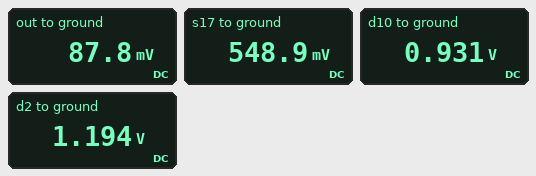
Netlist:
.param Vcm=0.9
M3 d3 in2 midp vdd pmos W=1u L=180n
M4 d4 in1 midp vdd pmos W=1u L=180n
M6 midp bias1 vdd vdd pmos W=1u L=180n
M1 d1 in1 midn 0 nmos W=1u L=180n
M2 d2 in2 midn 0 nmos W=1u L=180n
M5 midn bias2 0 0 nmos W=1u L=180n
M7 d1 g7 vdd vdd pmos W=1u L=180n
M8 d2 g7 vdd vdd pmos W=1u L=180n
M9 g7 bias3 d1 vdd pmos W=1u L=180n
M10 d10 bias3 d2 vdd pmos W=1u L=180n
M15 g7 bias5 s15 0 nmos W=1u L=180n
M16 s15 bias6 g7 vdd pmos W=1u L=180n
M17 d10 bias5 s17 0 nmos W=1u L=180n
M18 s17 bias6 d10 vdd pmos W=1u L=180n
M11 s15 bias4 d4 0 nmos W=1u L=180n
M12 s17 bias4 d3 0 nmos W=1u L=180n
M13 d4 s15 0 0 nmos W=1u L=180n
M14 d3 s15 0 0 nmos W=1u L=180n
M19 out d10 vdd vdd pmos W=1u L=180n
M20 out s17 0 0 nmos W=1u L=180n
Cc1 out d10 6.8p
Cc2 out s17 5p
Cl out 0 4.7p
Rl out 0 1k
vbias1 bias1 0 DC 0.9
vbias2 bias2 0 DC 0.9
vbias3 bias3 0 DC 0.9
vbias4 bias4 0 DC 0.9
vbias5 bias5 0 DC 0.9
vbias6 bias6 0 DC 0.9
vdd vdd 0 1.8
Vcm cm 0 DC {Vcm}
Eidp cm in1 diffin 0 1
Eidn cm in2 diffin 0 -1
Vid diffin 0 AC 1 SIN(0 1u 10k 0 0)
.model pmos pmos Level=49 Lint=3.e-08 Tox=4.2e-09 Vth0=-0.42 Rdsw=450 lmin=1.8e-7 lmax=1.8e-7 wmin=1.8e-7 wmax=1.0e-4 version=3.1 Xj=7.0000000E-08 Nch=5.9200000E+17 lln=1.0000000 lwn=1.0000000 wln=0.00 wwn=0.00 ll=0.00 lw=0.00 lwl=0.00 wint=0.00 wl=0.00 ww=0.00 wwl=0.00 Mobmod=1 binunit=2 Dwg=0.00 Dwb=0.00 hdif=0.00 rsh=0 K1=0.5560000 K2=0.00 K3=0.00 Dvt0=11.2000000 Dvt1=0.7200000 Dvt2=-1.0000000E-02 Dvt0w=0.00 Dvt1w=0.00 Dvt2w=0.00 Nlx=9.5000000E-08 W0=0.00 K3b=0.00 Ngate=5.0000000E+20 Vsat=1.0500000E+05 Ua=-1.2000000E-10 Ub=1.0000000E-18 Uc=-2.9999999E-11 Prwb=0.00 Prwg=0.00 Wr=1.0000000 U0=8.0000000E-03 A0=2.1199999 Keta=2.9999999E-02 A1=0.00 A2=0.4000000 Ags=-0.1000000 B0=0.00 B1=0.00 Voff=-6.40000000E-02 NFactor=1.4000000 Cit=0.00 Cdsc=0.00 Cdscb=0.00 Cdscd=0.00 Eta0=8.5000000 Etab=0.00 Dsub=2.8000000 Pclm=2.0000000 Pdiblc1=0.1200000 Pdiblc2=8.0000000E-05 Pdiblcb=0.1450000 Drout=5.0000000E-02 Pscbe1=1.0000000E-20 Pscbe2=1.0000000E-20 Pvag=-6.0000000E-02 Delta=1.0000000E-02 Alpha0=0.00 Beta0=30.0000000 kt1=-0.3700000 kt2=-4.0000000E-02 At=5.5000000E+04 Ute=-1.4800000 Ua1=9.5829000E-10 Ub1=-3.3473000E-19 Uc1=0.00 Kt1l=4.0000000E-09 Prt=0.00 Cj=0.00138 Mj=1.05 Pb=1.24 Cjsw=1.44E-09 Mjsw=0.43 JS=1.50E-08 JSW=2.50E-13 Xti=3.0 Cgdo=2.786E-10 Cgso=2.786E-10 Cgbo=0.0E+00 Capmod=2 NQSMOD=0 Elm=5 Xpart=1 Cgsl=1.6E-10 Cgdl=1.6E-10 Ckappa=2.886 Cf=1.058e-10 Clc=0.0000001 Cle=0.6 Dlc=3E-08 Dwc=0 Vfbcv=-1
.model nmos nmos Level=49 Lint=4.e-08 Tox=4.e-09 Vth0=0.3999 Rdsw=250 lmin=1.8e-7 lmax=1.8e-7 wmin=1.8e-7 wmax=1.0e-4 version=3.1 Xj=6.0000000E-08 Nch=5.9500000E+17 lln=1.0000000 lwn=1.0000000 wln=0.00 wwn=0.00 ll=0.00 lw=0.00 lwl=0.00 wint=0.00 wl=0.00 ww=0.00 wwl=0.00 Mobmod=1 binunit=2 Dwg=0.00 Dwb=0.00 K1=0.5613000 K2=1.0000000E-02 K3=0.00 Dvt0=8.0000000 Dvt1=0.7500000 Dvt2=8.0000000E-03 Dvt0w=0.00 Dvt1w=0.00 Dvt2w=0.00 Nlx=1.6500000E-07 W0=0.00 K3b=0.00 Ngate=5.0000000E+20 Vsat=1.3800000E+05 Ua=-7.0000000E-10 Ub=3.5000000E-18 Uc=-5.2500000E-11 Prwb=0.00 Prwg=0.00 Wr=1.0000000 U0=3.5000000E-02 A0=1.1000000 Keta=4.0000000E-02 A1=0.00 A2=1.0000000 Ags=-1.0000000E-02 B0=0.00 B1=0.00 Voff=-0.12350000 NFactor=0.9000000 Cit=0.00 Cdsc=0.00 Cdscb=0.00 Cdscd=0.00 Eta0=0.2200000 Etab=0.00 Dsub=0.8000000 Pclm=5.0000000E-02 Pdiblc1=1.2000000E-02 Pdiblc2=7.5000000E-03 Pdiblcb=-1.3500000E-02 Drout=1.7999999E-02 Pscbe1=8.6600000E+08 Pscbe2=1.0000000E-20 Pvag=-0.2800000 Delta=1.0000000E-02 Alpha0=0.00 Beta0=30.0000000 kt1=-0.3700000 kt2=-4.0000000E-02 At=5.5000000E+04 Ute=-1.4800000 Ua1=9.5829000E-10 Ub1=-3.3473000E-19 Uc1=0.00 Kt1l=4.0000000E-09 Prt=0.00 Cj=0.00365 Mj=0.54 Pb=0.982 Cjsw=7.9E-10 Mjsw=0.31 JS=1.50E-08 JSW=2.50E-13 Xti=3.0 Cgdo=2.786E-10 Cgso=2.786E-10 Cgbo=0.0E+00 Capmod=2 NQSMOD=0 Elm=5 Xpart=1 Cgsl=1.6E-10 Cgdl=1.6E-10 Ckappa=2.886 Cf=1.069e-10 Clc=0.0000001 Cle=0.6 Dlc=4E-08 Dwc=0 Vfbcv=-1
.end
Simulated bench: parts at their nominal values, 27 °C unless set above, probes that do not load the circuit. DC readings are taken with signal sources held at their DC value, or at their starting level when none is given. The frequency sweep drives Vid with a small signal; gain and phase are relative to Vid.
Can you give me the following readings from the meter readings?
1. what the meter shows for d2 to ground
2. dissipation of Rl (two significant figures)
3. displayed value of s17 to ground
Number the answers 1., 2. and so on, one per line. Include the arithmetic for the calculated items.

1. 1.194 V
2. (87.8 mV)^2 / 1 kΩ = 7.7 µW
3. 548.9 mV
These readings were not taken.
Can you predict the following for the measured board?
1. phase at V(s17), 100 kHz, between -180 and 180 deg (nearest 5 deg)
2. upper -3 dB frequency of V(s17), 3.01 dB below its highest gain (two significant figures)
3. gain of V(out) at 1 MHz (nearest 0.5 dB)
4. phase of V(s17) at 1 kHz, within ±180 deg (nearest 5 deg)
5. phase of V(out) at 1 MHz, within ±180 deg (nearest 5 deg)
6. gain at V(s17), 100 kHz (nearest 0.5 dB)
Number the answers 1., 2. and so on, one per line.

1. 150 deg
2. 4.9 kHz
3. -10.0 dB
4. 170 deg
5. -100 deg
6. 13.5 dB
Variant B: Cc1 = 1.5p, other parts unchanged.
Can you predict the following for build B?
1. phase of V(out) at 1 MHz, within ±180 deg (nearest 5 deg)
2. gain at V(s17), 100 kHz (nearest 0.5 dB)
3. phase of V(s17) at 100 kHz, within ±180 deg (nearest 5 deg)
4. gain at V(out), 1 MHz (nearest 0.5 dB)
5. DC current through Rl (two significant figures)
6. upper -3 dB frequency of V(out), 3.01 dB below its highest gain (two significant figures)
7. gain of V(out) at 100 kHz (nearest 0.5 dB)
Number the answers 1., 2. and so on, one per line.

1. -95 deg
2. 10.5 dB
3. 115 deg
4. -1.0 dB
5. 88 µA
6. 15 kHz
7. 19.5 dB
